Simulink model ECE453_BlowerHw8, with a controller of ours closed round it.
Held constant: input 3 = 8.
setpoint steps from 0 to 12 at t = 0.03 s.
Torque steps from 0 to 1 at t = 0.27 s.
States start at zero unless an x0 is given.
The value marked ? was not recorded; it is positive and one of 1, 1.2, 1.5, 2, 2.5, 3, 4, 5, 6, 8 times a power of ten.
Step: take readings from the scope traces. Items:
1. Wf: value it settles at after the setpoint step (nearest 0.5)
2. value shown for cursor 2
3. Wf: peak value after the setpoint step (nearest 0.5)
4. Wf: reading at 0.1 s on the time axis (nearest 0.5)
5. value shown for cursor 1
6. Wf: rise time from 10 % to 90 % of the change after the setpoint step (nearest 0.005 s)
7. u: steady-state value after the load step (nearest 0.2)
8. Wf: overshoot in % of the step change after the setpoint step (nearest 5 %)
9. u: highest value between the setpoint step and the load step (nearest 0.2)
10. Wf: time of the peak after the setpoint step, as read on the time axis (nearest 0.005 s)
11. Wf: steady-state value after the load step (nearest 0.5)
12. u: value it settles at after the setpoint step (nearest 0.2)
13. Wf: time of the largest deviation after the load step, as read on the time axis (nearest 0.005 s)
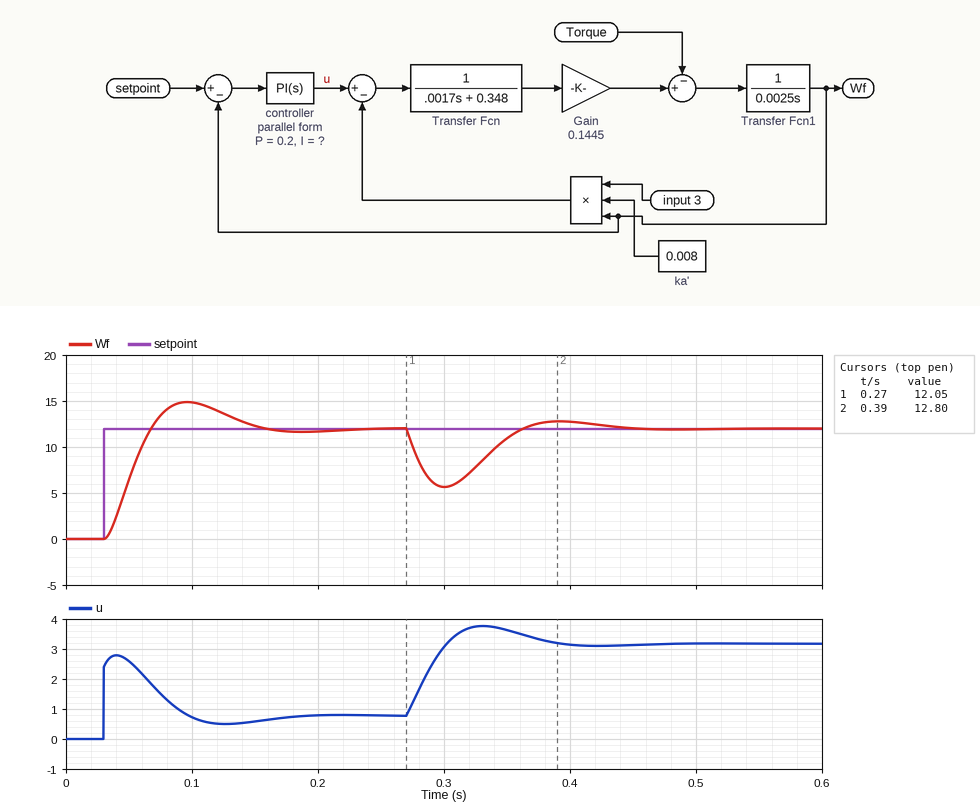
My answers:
12.0
12.80
15.0
15.0
12.05
0.025 s
3.2
25 %
2.8
0.095 s
12.0
0.8
0.300 s
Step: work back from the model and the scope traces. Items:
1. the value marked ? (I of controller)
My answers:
8
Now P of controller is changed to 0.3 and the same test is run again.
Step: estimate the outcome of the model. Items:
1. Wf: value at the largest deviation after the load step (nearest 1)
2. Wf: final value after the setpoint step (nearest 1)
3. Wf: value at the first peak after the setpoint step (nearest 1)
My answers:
7
12
14
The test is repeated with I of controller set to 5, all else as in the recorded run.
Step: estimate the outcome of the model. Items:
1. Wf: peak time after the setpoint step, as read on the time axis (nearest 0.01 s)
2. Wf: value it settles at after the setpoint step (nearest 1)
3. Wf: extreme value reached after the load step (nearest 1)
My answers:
0.11 s
12
5
